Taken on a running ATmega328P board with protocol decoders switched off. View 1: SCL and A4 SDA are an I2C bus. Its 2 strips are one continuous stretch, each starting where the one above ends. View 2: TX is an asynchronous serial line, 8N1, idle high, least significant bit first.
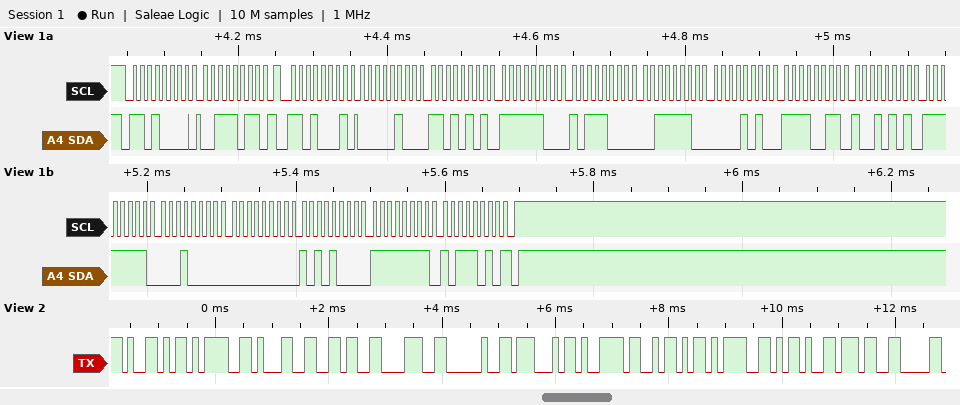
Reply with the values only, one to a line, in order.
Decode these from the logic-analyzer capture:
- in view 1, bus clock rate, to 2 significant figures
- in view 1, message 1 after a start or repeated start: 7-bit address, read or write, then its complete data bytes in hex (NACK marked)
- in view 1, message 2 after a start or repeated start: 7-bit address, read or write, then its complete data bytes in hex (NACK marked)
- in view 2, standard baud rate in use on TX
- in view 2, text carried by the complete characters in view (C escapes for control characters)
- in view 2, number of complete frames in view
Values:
100 kHz
0x68 write: 3B
0x68 read: 04 D5 FC B8 3E 0A F3 95 FF 10 00 A8 FF BA NACK
9600 baud
"Y=168 GyZ=-7"
12
